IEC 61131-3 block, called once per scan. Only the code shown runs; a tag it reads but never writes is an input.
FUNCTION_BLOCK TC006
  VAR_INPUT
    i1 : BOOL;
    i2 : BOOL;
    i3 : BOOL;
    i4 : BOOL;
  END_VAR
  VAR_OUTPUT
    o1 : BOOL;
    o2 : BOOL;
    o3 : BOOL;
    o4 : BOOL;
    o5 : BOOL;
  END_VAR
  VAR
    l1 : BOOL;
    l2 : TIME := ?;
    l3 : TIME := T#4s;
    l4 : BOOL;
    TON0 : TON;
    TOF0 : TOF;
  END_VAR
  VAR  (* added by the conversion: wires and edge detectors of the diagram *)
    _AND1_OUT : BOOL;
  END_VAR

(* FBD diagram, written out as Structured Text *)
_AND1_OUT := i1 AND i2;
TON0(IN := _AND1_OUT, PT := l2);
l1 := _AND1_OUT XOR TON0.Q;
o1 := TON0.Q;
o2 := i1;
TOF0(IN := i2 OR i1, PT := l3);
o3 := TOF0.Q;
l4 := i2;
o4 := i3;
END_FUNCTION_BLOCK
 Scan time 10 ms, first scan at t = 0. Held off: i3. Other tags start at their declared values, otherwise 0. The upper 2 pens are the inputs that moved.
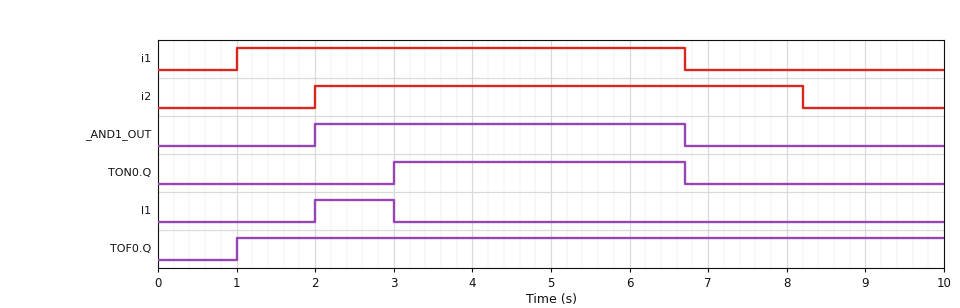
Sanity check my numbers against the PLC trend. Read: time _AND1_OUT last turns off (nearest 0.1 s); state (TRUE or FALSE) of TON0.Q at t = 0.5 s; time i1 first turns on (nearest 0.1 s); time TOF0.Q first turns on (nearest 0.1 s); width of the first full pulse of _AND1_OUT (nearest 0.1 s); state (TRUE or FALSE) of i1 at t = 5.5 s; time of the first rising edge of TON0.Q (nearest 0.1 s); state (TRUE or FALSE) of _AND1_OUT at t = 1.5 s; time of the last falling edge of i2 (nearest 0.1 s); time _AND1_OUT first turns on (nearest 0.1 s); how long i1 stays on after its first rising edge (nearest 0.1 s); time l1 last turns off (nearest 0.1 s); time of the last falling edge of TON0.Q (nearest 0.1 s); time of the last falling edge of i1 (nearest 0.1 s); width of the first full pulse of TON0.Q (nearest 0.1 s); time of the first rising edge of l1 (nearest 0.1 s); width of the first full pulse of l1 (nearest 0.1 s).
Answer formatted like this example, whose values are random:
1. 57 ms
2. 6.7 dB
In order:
1. 6.7 s
2. FALSE
3. 1.0 s
4. 1.0 s
5. 4.7 s
6. TRUE
7. 3.0 s
8. FALSE
9. 8.2 s
10. 2.0 s
11. 5.7 s
12. 3.0 s
13. 6.7 s
14. 6.7 s
15. 3.7 s
16. 2.0 s
17. 1.0 s
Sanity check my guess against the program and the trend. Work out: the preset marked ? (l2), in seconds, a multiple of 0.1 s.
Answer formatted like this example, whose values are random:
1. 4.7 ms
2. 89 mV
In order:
1. 1.0 s
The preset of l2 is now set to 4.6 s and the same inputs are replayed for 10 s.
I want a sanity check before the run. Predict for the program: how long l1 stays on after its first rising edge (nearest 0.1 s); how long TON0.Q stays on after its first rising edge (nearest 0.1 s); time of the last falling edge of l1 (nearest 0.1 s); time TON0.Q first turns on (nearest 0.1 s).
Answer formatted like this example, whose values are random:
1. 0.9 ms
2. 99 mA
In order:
1. 4.6 s
2. 0.1 s
3. 6.6 s
4. 6.6 s
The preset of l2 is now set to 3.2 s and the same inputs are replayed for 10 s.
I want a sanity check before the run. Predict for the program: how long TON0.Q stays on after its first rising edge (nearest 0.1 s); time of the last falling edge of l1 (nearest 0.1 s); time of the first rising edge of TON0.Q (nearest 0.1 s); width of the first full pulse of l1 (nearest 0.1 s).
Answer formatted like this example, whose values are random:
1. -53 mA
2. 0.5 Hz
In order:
1. 1.5 s
2. 5.2 s
3. 5.2 s
4. 3.2 s
